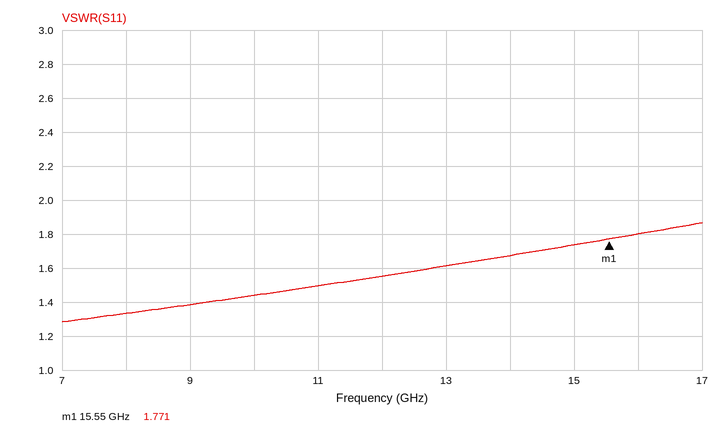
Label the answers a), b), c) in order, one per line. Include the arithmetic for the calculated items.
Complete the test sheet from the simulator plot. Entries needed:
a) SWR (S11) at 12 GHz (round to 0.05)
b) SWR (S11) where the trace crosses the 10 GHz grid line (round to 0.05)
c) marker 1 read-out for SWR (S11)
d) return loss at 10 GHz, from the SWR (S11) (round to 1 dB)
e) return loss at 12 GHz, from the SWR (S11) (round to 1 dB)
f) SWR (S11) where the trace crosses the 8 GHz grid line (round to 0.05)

a) 1.55
b) 1.45
c) 1.771
d) −20 log10((1.45 − 1)/(1.45 + 1)) ≈ 15 dB
e) −20 log10((1.55 − 1)/(1.55 + 1)) ≈ 13 dB
f) 1.35
